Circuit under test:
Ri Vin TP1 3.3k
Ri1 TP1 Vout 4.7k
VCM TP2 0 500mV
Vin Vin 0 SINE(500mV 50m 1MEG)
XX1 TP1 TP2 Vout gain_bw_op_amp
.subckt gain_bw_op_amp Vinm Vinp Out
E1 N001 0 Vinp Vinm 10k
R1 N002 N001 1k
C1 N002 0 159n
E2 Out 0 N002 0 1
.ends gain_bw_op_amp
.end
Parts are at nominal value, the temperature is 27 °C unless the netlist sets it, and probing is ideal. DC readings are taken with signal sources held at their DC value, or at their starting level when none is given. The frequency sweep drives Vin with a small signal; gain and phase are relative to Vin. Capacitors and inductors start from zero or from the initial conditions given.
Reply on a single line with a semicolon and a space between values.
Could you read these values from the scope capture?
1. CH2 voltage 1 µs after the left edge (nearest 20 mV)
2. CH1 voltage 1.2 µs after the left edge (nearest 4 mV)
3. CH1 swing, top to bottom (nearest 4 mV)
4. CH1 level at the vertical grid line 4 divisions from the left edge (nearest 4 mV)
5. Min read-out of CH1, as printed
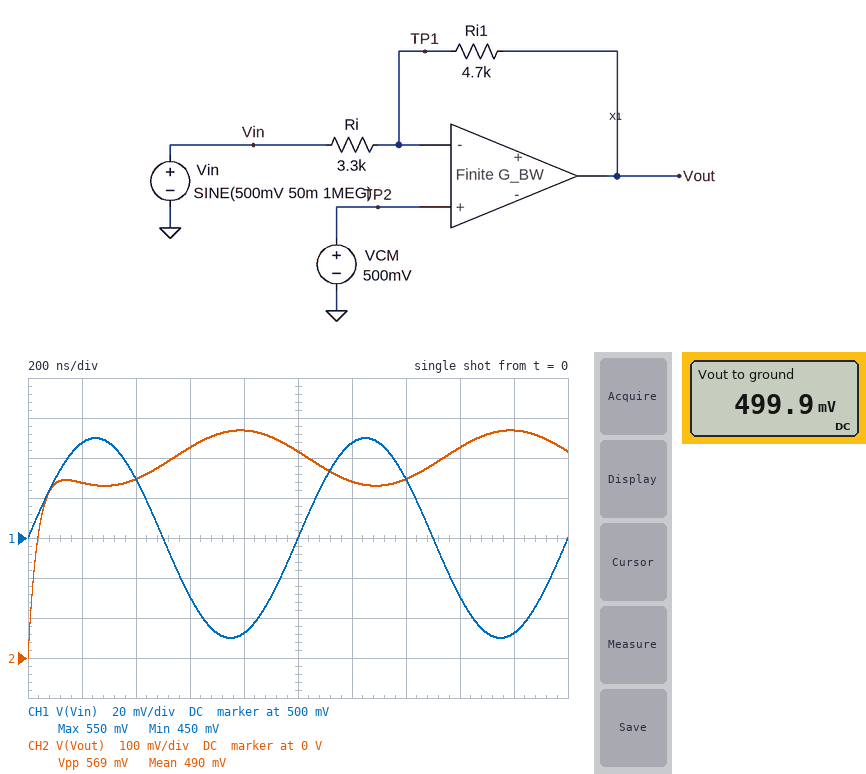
520 mV; 548 mV; 100 mV; 452 mV; 450 mV
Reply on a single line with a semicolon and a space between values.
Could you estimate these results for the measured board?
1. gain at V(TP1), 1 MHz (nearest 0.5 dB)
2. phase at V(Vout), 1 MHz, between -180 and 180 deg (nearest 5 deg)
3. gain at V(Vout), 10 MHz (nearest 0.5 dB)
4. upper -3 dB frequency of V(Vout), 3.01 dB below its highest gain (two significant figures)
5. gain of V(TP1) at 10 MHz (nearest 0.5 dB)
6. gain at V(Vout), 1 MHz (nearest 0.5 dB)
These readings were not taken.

-17.0 dB; 165 deg; -5.5 dB; 4.1 MHz; -5.5 dB; 3.0 dB
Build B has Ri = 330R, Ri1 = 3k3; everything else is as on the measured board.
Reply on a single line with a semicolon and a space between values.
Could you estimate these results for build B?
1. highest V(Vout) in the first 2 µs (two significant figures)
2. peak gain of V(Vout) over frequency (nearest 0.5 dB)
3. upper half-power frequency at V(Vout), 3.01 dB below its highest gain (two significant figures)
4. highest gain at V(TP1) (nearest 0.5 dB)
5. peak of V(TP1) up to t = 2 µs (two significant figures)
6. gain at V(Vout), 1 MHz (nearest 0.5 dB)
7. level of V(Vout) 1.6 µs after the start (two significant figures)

840 mV; 20.0 dB; 910 kHz; -1.0 dB; 530 mV; 16.5 dB; 430 mV
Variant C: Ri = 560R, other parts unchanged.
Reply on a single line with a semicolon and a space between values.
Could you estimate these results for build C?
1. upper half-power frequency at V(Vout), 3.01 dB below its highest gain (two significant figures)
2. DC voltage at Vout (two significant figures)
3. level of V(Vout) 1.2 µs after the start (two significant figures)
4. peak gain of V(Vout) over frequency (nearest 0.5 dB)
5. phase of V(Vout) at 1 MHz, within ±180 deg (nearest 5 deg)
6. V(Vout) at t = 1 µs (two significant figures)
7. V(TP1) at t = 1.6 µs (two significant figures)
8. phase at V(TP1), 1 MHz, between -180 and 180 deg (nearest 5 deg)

1.1 MHz; 500 mV; 350 mV; 18.5 dB; 135 deg; 710 mV; 470 mV; 45 deg
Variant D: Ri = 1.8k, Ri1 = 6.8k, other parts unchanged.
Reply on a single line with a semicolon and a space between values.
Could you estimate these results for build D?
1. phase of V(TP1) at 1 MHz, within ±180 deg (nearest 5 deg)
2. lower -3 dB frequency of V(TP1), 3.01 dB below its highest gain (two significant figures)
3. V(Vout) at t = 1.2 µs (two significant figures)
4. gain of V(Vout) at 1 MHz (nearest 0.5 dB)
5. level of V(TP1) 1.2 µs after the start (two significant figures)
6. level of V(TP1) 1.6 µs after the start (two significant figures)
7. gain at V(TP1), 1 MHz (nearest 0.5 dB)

65 deg; 2.1 MHz; 380 mV; 10.5 dB; 510 mV; 480 mV; -9.5 dB
